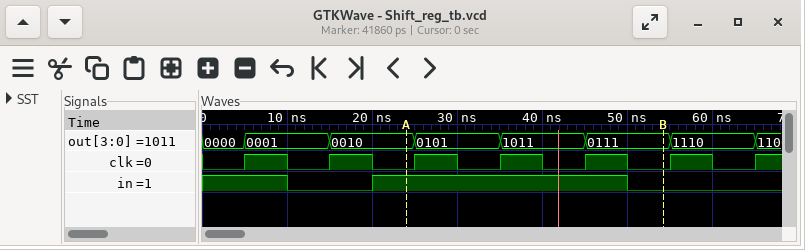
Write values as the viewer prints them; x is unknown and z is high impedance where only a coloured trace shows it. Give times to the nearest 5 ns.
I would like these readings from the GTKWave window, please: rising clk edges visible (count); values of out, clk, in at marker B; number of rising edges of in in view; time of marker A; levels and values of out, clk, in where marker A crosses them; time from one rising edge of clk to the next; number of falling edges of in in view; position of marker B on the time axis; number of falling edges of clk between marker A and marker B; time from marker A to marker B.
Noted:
7
out=0111, clk=0, in=0
1
25 ns
out=0010, clk=0, in=1
10 ns
2
55 ns
3
30 ns
